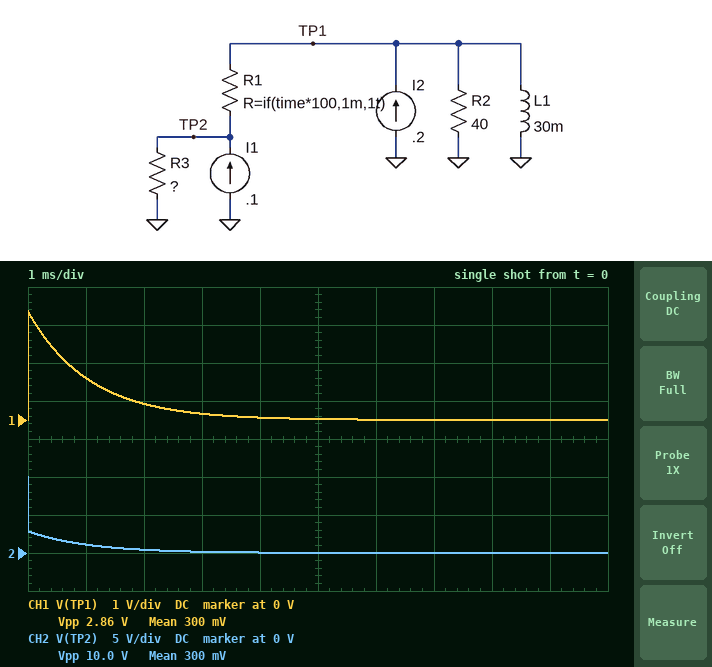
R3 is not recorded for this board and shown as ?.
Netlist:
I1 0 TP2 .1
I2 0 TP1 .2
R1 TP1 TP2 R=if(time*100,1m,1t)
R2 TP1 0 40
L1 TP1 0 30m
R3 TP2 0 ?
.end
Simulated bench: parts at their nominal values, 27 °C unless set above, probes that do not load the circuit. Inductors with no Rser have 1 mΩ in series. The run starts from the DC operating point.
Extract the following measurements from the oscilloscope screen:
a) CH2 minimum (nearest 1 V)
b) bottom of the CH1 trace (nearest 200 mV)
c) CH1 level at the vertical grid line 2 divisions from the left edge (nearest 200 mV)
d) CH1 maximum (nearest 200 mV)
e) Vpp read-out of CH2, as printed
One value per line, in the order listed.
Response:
0 V
0 V
400 mV
2.8 V
10.0 V
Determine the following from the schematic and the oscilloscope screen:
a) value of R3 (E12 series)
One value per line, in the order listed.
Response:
100 Ω
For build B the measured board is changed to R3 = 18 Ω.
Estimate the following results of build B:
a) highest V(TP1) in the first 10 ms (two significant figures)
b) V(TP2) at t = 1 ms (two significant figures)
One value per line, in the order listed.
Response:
1.2 V
820 mV
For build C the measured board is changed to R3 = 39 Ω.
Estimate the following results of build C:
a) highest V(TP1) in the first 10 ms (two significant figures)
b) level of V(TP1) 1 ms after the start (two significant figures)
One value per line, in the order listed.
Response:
2.0 V
1.0 V
